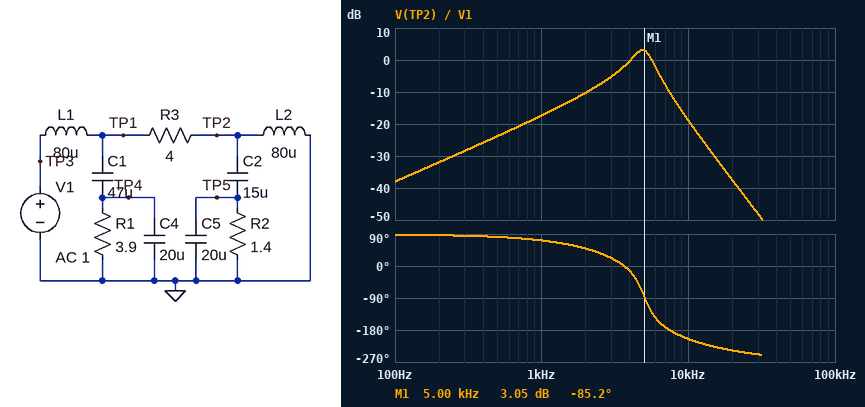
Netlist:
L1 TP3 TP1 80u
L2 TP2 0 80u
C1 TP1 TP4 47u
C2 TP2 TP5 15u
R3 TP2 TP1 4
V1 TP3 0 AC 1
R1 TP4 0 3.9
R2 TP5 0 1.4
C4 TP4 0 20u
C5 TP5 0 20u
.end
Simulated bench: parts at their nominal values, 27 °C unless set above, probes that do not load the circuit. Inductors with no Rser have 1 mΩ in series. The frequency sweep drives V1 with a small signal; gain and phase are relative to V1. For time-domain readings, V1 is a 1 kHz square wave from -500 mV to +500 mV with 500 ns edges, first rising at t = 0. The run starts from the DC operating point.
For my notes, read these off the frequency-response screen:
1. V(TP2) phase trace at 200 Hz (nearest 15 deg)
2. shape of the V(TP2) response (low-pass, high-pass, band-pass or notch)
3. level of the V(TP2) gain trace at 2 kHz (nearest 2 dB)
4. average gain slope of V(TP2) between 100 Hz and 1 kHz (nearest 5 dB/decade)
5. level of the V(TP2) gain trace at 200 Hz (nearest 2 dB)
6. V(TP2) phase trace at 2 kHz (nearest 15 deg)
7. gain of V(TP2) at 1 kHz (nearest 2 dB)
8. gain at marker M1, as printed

90 deg
band-pass
-10 dB
20 dB/decade
-32 dB
45 deg
-18 dB
3.05 dB
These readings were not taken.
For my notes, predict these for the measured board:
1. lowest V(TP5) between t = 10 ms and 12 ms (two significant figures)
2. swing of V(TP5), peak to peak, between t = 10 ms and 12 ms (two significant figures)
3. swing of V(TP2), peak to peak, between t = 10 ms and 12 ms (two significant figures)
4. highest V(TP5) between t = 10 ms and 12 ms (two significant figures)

-110 mV
230 mV
810 mV
110 mV
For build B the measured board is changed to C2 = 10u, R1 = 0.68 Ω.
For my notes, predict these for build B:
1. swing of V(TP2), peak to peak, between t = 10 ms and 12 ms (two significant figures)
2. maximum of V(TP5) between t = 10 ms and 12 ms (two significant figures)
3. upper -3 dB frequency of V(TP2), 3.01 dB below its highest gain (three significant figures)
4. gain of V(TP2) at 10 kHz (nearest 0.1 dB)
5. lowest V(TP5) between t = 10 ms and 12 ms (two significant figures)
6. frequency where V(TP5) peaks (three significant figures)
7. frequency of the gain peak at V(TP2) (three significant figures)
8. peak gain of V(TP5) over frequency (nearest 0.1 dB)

580 mV
48 mV
5.60 kHz
-20.2 dB
-48 mV
4.12 kHz
3.26 kHz
-17.7 dB
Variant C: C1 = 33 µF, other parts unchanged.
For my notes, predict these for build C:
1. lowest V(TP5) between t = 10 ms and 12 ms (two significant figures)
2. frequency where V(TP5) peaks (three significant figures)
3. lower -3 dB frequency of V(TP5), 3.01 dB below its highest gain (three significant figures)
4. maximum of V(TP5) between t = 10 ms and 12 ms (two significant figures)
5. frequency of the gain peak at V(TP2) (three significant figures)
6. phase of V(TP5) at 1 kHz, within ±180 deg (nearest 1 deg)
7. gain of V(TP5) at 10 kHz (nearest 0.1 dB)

-130 mV
5.11 kHz
4.40 kHz
130 mV
5.08 kHz
146 deg
-25.5 dB
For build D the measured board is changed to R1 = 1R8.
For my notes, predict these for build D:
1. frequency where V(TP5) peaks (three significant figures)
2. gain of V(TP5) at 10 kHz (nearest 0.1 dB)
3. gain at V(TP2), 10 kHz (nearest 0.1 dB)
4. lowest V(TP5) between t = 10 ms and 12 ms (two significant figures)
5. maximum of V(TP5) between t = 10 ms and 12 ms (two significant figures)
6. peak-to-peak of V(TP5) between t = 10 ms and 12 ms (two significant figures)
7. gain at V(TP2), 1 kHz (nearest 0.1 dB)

4.71 kHz
-27.5 dB
-19.7 dB
-80 mV
80 mV
160 mV
-17.0 dB
